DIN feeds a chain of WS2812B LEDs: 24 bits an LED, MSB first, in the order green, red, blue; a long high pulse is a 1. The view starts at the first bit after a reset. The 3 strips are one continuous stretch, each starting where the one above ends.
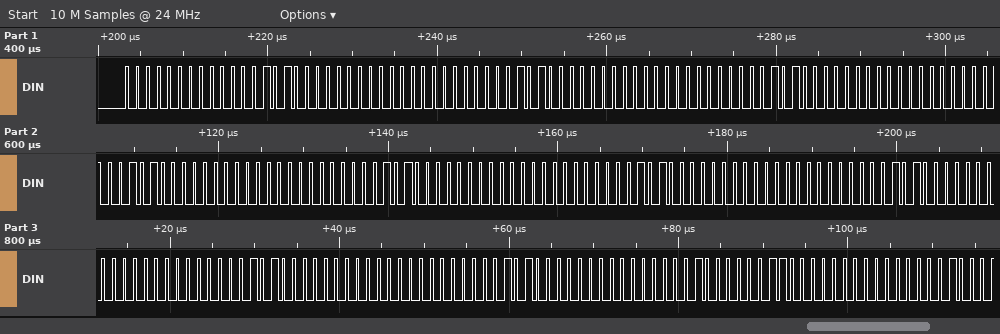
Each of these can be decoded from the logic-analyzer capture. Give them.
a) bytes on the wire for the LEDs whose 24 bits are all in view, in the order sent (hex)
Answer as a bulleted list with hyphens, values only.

- 00 05 00 00 05 00 00 05 00 00 05 00 00 05 00 00 05 00 00 05 00 00 05 00 00 05 00 01 03 00
